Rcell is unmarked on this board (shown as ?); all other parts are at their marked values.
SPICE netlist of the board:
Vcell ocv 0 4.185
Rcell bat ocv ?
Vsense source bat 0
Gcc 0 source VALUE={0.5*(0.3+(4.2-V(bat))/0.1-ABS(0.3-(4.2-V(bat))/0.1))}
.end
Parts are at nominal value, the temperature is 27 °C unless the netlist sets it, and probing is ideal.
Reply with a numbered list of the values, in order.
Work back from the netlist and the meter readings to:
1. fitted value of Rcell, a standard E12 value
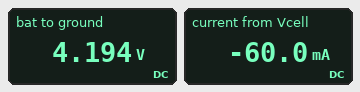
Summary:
1. 0.15 Ω
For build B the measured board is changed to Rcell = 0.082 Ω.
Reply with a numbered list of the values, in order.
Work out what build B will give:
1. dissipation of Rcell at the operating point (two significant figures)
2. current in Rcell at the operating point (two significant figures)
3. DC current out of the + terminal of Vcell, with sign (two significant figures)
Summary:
1. 560 µW
2. 82 mA
3. -82 mA
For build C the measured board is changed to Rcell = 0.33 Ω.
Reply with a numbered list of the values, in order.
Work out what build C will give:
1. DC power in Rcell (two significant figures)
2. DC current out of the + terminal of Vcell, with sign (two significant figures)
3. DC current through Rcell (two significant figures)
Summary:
1. 400 µW
2. -35 mA
3. 35 mA
